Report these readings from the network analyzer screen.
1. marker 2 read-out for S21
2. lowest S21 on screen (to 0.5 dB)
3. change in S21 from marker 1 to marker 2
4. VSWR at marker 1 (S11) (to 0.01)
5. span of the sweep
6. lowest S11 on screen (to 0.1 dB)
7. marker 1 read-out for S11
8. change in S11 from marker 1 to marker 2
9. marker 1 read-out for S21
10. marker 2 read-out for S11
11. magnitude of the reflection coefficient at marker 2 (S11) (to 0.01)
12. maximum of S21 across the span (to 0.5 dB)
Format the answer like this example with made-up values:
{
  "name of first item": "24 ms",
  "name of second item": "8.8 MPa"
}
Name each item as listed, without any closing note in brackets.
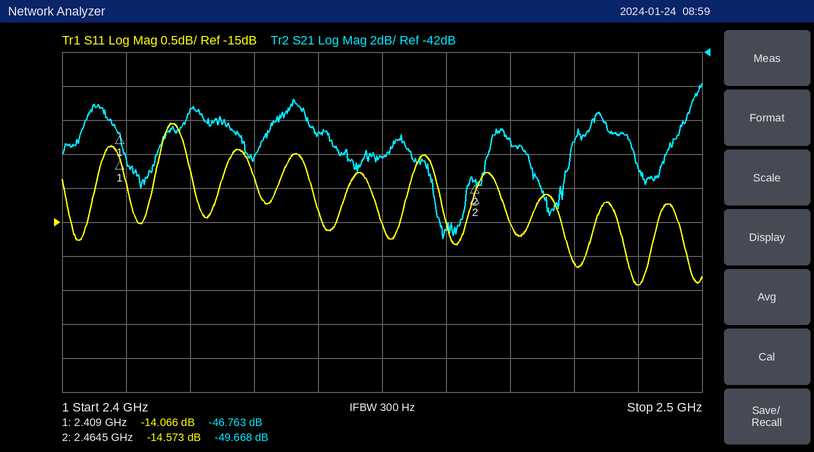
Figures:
{
  "marker 2 read-out for S21": "-49.668 dB",
  "lowest S21 on screen": "-53.0 dB",
  "change in S21 from marker 1 to marker 2": "-2.905 dB",
  "VSWR at marker 1 (S11)": "1.49",
  "span of the sweep": "100 MHz",
  "lowest S11 on screen": "-15.9 dB",
  "marker 1 read-out for S11": "-14.066 dB",
  "change in S11 from marker 1 to marker 2": "-0.507 dB",
  "marker 1 read-out for S21": "-46.763 dB",
  "marker 2 read-out for S11": "-14.573 dB",
  "magnitude of the reflection coefficient at marker 2 (S11)": "0.19",
  "maximum of S21 across the span": "-44.0 dB"
}
